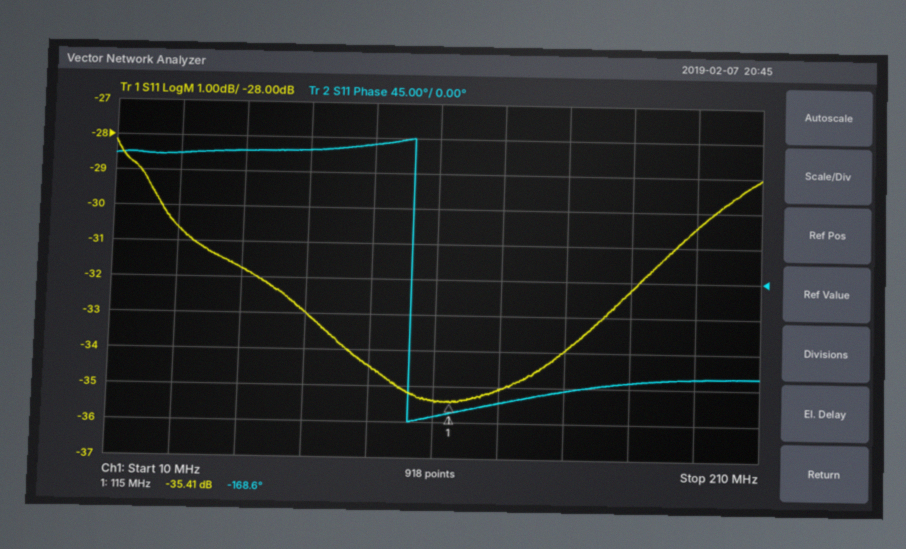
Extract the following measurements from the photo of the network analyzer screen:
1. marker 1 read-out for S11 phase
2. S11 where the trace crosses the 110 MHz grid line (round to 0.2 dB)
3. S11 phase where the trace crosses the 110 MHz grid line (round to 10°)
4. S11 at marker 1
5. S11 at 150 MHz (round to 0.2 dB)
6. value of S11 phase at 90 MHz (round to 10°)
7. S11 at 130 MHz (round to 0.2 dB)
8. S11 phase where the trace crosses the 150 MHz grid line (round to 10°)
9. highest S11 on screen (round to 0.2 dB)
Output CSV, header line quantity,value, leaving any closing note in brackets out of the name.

quantity,value
marker 1 read-out for S11 phase,-168.6°
S11 where the trace crosses the 110 MHz grid line,-35.4 dB
S11 phase where the trace crosses the 110 MHz grid line,-170°
S11 at marker 1,-35.41 dB
S11 at 150 MHz,-34.0 dB
value of S11 phase at 90 MHz,170°
S11 at 130 MHz,-35.0 dB
S11 phase where the trace crosses the 150 MHz grid line,-140°
highest S11 on screen,-28.2 dB
